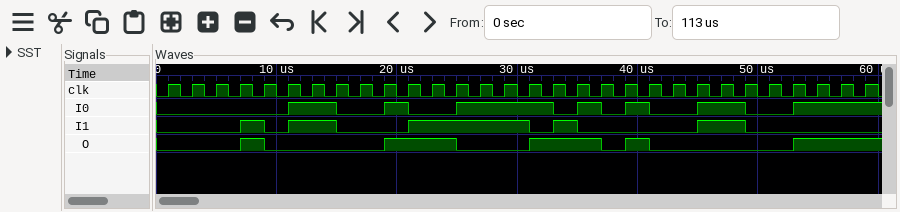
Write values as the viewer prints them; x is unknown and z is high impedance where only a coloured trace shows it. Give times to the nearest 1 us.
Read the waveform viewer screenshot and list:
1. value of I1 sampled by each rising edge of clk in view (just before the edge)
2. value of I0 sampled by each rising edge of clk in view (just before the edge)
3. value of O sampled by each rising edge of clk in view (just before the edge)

0 0 0 0 1 0 1 1 0 0 0 1 1 1 1 1 0 1 0 0 0 0 0 1 1 0 0 0 0 0
0 0 0 0 0 0 1 1 0 0 1 0 0 1 1 1 1 0 1 0 1 0 0 1 1 0 0 1 1 1
0 0 0 0 1 0 0 0 0 0 1 1 1 0 0 0 1 1 1 0 1 0 0 0 0 0 0 1 1 1
